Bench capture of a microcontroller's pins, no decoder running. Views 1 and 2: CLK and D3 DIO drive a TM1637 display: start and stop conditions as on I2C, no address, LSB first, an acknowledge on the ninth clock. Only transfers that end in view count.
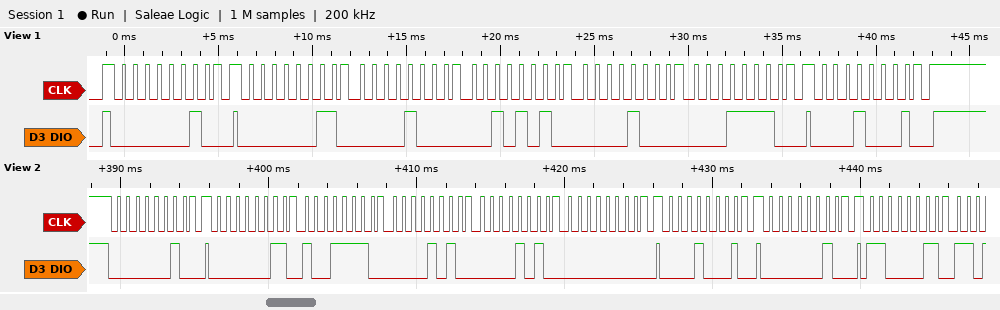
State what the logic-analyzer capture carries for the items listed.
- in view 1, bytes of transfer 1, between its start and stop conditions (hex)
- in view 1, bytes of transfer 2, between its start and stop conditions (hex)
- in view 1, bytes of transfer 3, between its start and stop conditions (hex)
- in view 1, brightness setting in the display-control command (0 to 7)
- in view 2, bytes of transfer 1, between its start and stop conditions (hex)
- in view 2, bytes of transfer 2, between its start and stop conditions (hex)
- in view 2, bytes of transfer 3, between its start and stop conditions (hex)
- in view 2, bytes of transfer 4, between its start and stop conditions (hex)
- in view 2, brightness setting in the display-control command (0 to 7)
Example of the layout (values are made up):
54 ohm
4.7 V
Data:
40
C0 10 54 10 78
88
0
40
C0 79 50 50 00
88
40
0
